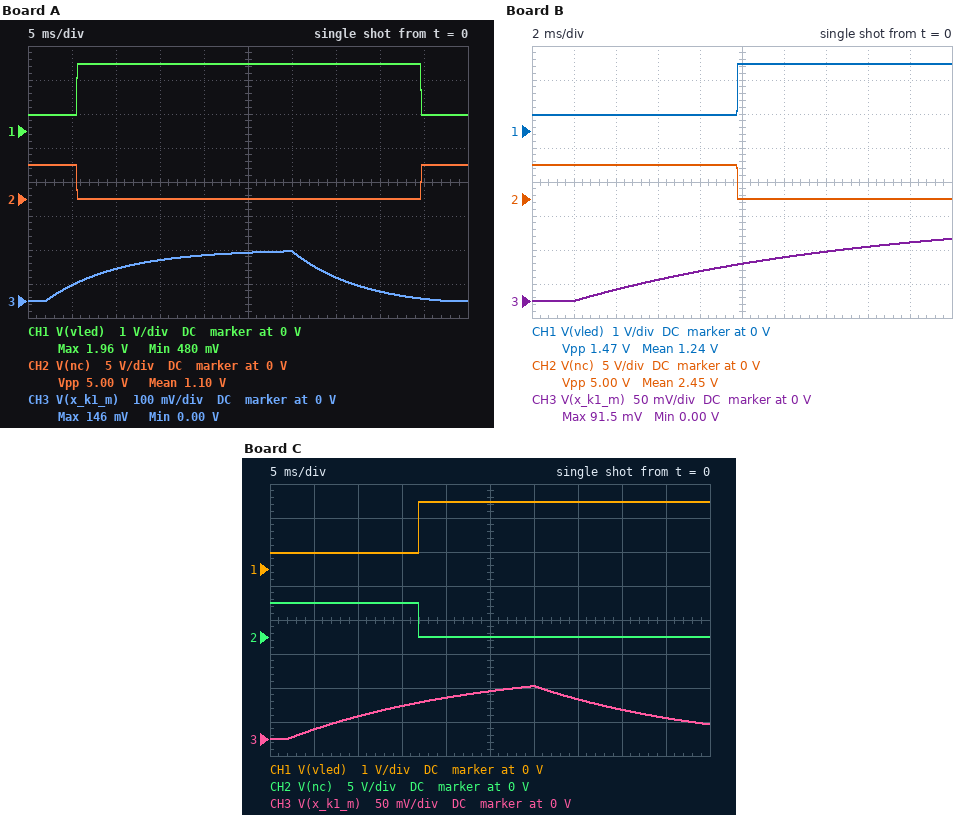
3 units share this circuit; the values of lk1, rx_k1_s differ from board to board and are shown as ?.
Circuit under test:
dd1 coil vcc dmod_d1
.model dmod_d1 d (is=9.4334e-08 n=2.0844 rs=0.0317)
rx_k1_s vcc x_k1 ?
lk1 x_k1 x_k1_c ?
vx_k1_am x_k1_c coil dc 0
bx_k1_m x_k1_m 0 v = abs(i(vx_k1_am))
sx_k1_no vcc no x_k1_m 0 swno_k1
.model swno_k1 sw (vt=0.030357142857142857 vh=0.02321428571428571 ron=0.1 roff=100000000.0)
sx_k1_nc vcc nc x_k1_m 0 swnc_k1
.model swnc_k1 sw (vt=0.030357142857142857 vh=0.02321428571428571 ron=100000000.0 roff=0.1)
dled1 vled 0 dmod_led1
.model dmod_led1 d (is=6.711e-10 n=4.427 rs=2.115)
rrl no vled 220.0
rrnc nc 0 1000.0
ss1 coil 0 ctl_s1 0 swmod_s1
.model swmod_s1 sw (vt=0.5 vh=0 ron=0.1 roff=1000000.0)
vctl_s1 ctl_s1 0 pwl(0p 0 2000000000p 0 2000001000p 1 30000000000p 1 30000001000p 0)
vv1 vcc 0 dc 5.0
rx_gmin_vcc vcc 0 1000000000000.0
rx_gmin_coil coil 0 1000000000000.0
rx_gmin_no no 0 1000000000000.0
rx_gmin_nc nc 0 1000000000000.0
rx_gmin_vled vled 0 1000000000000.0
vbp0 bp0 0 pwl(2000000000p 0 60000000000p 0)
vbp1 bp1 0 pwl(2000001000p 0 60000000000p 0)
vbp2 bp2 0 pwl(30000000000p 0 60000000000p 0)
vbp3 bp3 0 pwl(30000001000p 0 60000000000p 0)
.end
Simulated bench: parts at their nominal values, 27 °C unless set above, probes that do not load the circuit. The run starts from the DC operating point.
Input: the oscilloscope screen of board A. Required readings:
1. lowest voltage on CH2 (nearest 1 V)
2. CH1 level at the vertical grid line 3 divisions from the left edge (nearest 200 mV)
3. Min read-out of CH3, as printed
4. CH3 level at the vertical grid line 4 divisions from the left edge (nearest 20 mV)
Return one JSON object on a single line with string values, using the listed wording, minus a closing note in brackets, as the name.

{"lowest voltage on CH2": "0 V", "CH1 level at the vertical grid line 3 divisions from the left edge": "2.0 V", "Min read-out of CH3, as printed": "0.00 V", "CH3 level at the vertical grid line 4 divisions from the left edge": "140 mV"}
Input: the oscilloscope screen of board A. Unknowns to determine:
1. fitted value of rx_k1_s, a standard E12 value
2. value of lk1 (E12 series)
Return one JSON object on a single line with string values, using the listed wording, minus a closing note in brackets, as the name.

{"fitted value of rx_k1_s, a standard E12 value": "33 Ω", "value of lk1": "270 mH"}
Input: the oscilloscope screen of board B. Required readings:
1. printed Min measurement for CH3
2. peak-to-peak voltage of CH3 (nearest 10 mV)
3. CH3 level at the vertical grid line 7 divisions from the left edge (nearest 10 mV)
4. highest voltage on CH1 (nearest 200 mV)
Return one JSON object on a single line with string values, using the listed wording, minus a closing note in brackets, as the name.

{"printed Min measurement for CH3": "0.00 V", "peak-to-peak voltage of CH3": "90 mV", "CH3 level at the vertical grid line 7 divisions from the left edge": "70 mV", "highest voltage on CH1": "2.0 V"}
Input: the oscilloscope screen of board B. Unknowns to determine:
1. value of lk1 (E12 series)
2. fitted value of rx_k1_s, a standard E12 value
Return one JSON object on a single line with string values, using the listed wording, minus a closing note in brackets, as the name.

{"value of lk1": "560 mH", "fitted value of rx_k1_s, a standard E12 value": "39 Ω"}
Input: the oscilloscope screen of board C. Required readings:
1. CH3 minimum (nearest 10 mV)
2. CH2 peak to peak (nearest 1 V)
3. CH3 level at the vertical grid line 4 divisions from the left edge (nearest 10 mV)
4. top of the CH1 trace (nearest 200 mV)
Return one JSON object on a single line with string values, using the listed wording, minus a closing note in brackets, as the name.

{"CH3 minimum": "0 V", "CH2 peak to peak": "5 V", "CH3 level at the vertical grid line 4 divisions from the left edge": "60 mV", "top of the CH1 trace": "2.0 V"}
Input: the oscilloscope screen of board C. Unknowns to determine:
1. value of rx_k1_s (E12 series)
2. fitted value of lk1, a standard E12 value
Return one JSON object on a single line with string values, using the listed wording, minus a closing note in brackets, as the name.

{"value of rx_k1_s": "47 Ω", "fitted value of lk1, a standard E12 value": "1 H"}
